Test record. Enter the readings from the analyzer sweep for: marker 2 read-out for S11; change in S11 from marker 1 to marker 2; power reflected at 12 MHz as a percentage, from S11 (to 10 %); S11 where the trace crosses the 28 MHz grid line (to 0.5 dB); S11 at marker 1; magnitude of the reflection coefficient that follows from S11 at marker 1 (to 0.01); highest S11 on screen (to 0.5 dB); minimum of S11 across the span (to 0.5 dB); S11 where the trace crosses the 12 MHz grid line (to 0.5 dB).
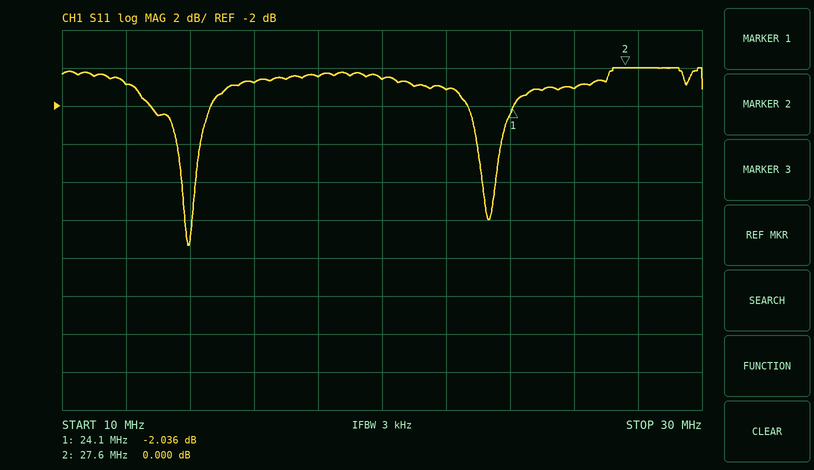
0.000 dB
2.036 dB
80 %
0.0 dB
-2.036 dB
0.79
0.0 dB
-9.5 dB
-1.0 dB
